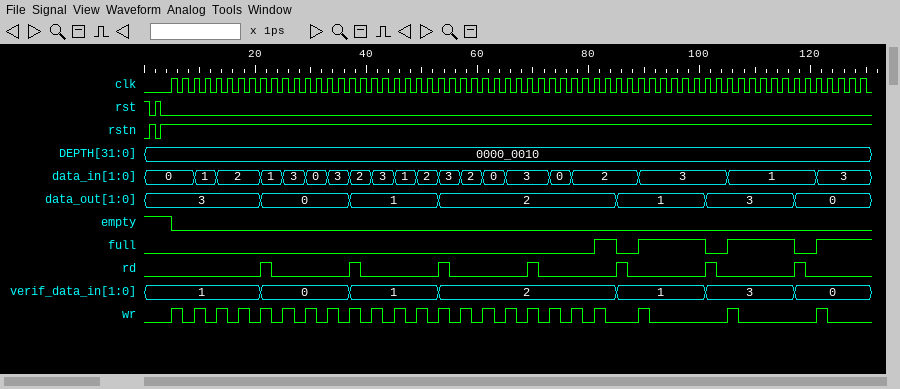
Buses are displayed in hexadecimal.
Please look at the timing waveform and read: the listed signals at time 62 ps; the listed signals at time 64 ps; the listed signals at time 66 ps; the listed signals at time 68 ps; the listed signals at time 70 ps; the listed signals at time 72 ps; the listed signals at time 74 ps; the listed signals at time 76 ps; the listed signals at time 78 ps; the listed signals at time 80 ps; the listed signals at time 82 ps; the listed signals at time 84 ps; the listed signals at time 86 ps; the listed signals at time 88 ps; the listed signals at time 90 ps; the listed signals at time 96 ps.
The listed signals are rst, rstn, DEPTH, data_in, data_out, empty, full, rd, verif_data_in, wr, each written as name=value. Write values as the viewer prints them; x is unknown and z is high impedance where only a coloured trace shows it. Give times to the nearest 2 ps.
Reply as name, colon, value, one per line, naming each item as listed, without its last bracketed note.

the listed signals at time 62 ps: rst=0, rstn=1, DEPTH=0000_0010, data_in=0, data_out=2, empty=0, full=0, rd=0, verif_data_in=2, wr=1
the listed signals at time 64 ps: rst=0, rstn=1, DEPTH=0000_0010, data_in=0, data_out=2, empty=0, full=0, rd=0, verif_data_in=2, wr=0
the listed signals at time 66 ps: rst=0, rstn=1, DEPTH=0000_0010, data_in=3, data_out=2, empty=0, full=0, rd=0, verif_data_in=2, wr=1
the listed signals at time 68 ps: rst=0, rstn=1, DEPTH=0000_0010, data_in=3, data_out=2, empty=0, full=0, rd=0, verif_data_in=2, wr=0
the listed signals at time 70 ps: rst=0, rstn=1, DEPTH=0000_0010, data_in=3, data_out=2, empty=0, full=0, rd=1, verif_data_in=2, wr=1
the listed signals at time 72 ps: rst=0, rstn=1, DEPTH=0000_0010, data_in=3, data_out=2, empty=0, full=0, rd=0, verif_data_in=2, wr=0
the listed signals at time 74 ps: rst=0, rstn=1, DEPTH=0000_0010, data_in=0, data_out=2, empty=0, full=0, rd=0, verif_data_in=2, wr=1
the listed signals at time 76 ps: rst=0, rstn=1, DEPTH=0000_0010, data_in=0, data_out=2, empty=0, full=0, rd=0, verif_data_in=2, wr=0
the listed signals at time 78 ps: rst=0, rstn=1, DEPTH=0000_0010, data_in=2, data_out=2, empty=0, full=0, rd=0, verif_data_in=2, wr=1
the listed signals at time 80 ps: rst=0, rstn=1, DEPTH=0000_0010, data_in=2, data_out=2, empty=0, full=0, rd=0, verif_data_in=2, wr=0
the listed signals at time 82 ps: rst=0, rstn=1, DEPTH=0000_0010, data_in=2, data_out=2, empty=0, full=1, rd=0, verif_data_in=2, wr=1
the listed signals at time 84 ps: rst=0, rstn=1, DEPTH=0000_0010, data_in=2, data_out=2, empty=0, full=1, rd=0, verif_data_in=2, wr=0
the listed signals at time 86 ps: rst=0, rstn=1, DEPTH=0000_0010, data_in=2, data_out=1, empty=0, full=0, rd=1, verif_data_in=1, wr=0
the listed signals at time 88 ps: rst=0, rstn=1, DEPTH=0000_0010, data_in=2, data_out=1, empty=0, full=0, rd=0, verif_data_in=1, wr=0
the listed signals at time 90 ps: rst=0, rstn=1, DEPTH=0000_0010, data_in=3, data_out=1, empty=0, full=1, rd=0, verif_data_in=1, wr=1
the listed signals at time 96 ps: rst=0, rstn=1, DEPTH=0000_0010, data_in=3, data_out=1, empty=0, full=1, rd=0, verif_data_in=1, wr=0
